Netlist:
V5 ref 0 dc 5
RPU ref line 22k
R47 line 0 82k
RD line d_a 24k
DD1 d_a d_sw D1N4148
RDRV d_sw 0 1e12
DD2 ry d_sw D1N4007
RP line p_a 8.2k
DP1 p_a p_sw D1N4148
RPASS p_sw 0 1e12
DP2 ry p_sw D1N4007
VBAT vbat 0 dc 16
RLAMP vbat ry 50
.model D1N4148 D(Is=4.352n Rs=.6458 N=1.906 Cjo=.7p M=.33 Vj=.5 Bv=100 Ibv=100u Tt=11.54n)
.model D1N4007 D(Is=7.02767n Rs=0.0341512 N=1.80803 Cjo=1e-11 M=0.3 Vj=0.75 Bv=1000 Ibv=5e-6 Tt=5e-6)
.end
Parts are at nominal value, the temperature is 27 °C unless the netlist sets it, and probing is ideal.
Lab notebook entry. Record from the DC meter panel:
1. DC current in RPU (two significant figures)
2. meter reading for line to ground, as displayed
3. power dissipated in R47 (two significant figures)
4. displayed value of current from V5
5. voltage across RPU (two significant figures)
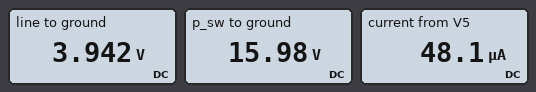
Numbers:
48 µA
3.942 V
190 µW
48.1 µA
1.1 V
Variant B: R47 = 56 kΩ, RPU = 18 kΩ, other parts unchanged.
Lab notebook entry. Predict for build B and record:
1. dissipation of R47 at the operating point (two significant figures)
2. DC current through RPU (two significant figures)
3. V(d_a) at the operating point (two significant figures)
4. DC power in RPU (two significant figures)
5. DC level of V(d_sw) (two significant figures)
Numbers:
260 µW
68 µA
3.8 V
82 µW
16 V
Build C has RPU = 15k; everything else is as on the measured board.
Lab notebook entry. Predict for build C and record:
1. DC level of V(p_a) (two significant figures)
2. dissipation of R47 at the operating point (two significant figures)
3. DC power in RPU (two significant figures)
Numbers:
4.2 V
220 µW
40 µW
